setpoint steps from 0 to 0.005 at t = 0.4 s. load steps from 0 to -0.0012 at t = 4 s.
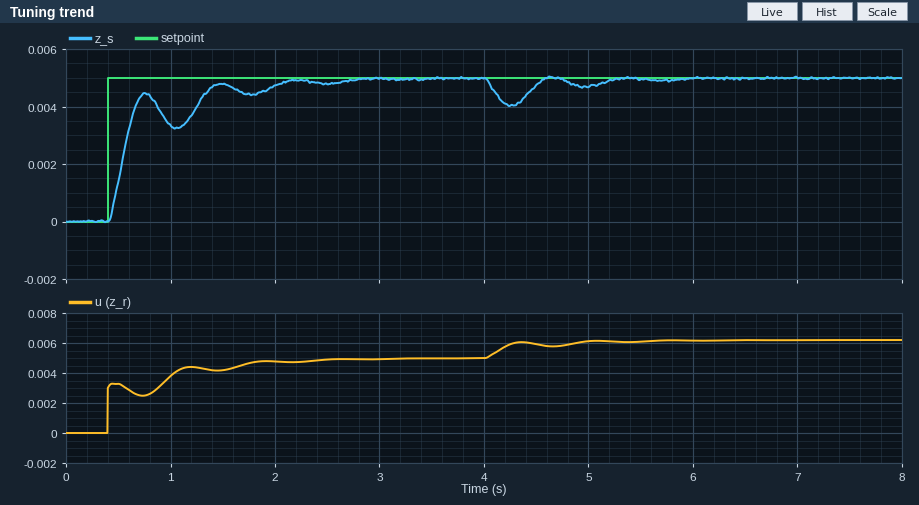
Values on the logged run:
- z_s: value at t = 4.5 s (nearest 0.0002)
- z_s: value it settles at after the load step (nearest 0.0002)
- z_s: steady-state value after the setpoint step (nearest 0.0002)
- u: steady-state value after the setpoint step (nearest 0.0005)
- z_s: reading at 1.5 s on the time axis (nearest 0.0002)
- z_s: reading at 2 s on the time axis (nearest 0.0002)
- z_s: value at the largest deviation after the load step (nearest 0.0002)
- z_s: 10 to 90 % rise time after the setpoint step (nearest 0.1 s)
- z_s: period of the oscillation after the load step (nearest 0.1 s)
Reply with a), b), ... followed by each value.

a) 0.0048
b) 0.0050
c) 0.0050
d) 0.0050
e) 0.0048
f) 0.0048
g) 0.0040
h) 0.9 s
i) 0.7 s
